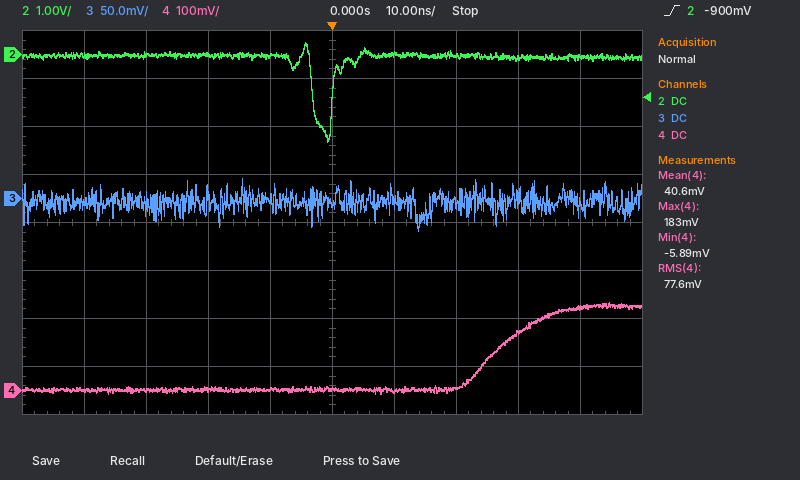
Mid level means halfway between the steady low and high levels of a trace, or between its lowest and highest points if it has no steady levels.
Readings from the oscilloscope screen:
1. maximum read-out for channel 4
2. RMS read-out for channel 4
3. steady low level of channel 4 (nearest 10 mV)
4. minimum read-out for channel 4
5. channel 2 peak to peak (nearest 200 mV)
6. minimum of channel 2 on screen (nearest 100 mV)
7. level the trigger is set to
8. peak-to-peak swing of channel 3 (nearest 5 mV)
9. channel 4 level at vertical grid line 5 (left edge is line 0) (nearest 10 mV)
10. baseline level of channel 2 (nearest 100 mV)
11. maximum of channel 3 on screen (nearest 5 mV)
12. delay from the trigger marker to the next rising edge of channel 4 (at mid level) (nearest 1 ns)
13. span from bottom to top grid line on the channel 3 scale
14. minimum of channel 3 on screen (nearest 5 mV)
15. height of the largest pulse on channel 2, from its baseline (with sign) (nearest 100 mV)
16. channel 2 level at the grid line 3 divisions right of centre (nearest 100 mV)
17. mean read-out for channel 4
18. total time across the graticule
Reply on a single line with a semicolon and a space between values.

183 mV; 77.6 mV; 0 mV; -5.89 mV; 2.0 V; -1.8 V; -900 mV; 55 mV; 0 mV; 0.0 V; 20 mV; 27 ns; 400 mV; -35 mV; -1.8 V; -100 mV; 40.6 mV; 100 ns
